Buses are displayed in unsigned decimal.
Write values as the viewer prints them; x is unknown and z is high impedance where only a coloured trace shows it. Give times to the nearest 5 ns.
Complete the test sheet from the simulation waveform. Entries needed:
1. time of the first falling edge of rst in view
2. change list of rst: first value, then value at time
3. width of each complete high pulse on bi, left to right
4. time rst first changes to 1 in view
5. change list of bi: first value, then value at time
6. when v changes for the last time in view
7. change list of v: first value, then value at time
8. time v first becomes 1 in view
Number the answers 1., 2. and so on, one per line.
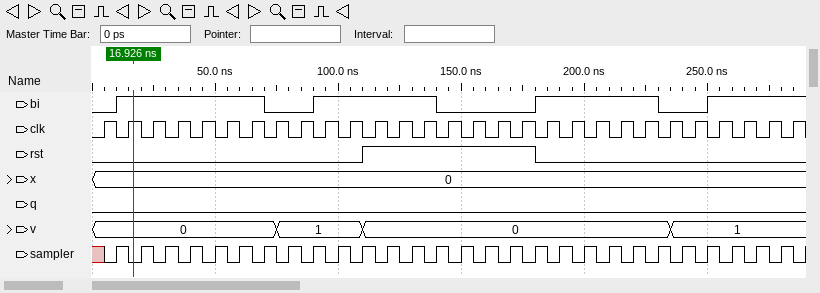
1. 180 ns
2. 0, 1 at 110 ns, 0 at 180 ns
3. 60 ns, 50 ns, 50 ns
4. 110 ns
5. 0, 1 at 10 ns, 0 at 70 ns, 1 at 90 ns, 0 at 140 ns, 1 at 180 ns, 0 at 230 ns, 1 at 250 ns
6. 235 ns
7. 0, 1 at 75 ns, 0 at 110 ns, 1 at 235 ns
8. 75 ns
